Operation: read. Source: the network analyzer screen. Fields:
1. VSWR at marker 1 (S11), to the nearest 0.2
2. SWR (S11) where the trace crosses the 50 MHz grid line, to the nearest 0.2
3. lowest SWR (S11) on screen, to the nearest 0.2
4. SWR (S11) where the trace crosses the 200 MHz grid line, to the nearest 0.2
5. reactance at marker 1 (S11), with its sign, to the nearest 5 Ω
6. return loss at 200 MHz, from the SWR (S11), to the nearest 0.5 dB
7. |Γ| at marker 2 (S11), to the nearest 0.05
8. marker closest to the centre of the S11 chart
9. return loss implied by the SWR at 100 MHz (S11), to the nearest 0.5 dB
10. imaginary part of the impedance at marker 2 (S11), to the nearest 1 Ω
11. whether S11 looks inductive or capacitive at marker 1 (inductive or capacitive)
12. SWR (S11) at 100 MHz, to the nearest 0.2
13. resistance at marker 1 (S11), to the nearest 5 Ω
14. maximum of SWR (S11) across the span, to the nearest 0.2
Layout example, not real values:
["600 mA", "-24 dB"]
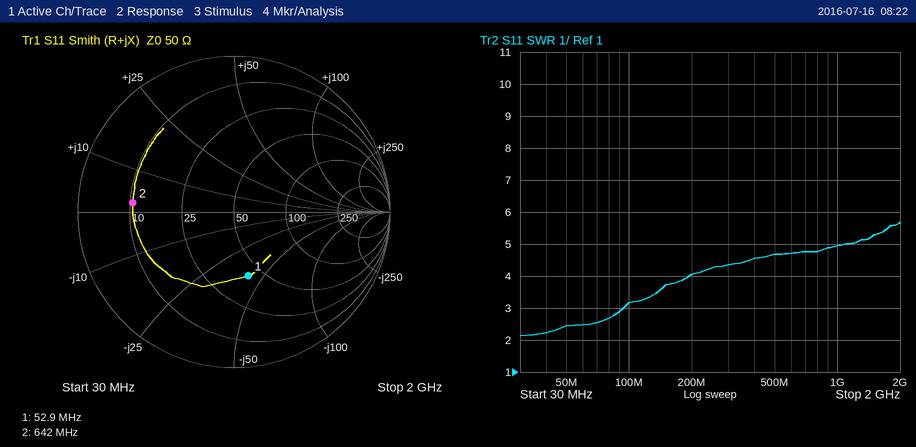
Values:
["2.4", "2.4", "2.2", "4.0", "-40 Ω", "4.5 dB", "0.65", "marker 1", "5.5 dB", "+2 Ω", "capacitive", "3.2", "40 Ω", "5.6"]
